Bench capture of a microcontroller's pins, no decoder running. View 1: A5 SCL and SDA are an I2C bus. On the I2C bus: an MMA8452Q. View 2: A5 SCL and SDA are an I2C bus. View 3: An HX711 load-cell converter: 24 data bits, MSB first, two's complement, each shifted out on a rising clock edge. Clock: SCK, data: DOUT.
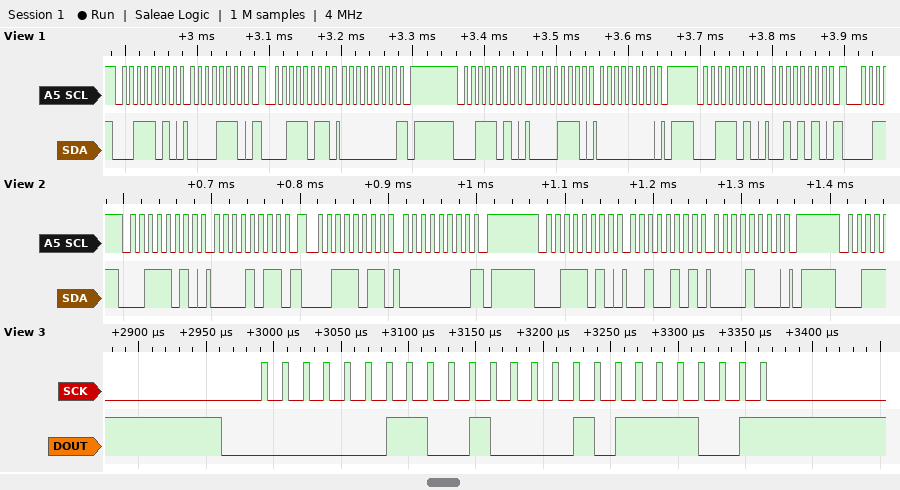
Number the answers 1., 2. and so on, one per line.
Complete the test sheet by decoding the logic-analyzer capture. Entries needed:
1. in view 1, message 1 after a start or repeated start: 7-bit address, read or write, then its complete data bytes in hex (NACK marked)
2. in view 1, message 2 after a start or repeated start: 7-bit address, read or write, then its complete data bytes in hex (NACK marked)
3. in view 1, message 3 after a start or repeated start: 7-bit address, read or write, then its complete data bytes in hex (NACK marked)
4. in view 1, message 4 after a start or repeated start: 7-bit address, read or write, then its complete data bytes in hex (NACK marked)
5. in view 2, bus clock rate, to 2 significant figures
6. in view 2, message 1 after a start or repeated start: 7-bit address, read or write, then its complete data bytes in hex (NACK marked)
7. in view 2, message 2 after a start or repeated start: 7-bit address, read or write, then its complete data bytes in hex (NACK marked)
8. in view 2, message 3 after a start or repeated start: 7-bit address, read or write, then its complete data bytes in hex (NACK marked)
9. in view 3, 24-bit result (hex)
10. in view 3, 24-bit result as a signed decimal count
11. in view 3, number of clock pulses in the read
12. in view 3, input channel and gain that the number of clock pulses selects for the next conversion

1. 0x1D write: 0E
2. 0x1D read: 00 NACK
3. 0x1D write: 0E 00
4. 0x1D write: 2A
5. 100 kHz
6. 0x1D write: 0B
7. 0x1D read: 00 NACK
8. 0x1D write: 25 08
9. 0x032179
10. 205177
11. 25
12. channel A, gain 128
